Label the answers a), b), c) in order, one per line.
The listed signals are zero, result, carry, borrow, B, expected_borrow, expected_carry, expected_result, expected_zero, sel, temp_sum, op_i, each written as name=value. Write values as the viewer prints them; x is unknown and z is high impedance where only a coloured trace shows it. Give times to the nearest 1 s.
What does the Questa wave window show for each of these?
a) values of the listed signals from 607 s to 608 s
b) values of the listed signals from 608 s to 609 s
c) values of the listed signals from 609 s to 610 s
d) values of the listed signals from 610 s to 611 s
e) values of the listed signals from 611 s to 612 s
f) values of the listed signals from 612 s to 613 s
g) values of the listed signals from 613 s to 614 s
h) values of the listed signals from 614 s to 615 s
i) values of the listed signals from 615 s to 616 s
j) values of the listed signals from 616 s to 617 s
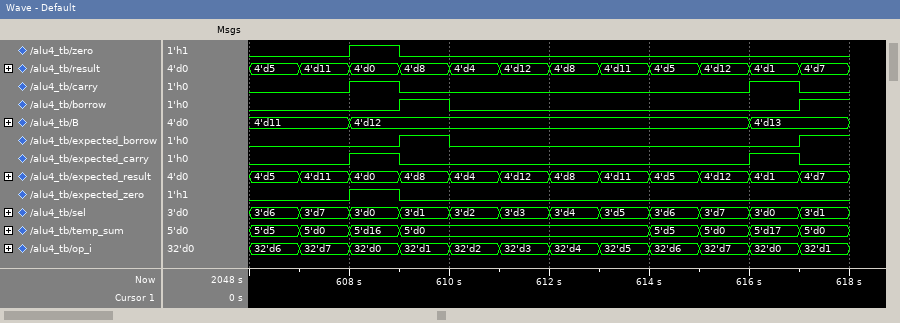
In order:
a) zero=0, result=4'd11, carry=0, borrow=0, B=4'd11, expected_borrow=0, expected_carry=0, expected_result=4'd11, expected_zero=0, sel=3'd7, temp_sum=5'd0, op_i=32'd7
b) zero=1, result=4'd0, carry=1, borrow=0, B=4'd12, expected_borrow=0, expected_carry=1, expected_result=4'd0, expected_zero=1, sel=3'd0, temp_sum=5'd16, op_i=32'd0
c) zero=0, result=4'd8, carry=0, borrow=1, B=4'd12, expected_borrow=1, expected_carry=0, expected_result=4'd8, expected_zero=0, sel=3'd1, temp_sum=5'd0, op_i=32'd1
d) zero=0, result=4'd4, carry=0, borrow=0, B=4'd12, expected_borrow=0, expected_carry=0, expected_result=4'd4, expected_zero=0, sel=3'd2, temp_sum=5'd0, op_i=32'd2
e) zero=0, result=4'd12, carry=0, borrow=0, B=4'd12, expected_borrow=0, expected_carry=0, expected_result=4'd12, expected_zero=0, sel=3'd3, temp_sum=5'd0, op_i=32'd3
f) zero=0, result=4'd8, carry=0, borrow=0, B=4'd12, expected_borrow=0, expected_carry=0, expected_result=4'd8, expected_zero=0, sel=3'd4, temp_sum=5'd0, op_i=32'd4
g) zero=0, result=4'd11, carry=0, borrow=0, B=4'd12, expected_borrow=0, expected_carry=0, expected_result=4'd11, expected_zero=0, sel=3'd5, temp_sum=5'd0, op_i=32'd5
h) zero=0, result=4'd5, carry=0, borrow=0, B=4'd12, expected_borrow=0, expected_carry=0, expected_result=4'd5, expected_zero=0, sel=3'd6, temp_sum=5'd5, op_i=32'd6
i) zero=0, result=4'd12, carry=0, borrow=0, B=4'd12, expected_borrow=0, expected_carry=0, expected_result=4'd12, expected_zero=0, sel=3'd7, temp_sum=5'd0, op_i=32'd7
j) zero=0, result=4'd1, carry=1, borrow=0, B=4'd13, expected_borrow=0, expected_carry=1, expected_result=4'd1, expected_zero=0, sel=3'd0, temp_sum=5'd17, op_i=32'd0
